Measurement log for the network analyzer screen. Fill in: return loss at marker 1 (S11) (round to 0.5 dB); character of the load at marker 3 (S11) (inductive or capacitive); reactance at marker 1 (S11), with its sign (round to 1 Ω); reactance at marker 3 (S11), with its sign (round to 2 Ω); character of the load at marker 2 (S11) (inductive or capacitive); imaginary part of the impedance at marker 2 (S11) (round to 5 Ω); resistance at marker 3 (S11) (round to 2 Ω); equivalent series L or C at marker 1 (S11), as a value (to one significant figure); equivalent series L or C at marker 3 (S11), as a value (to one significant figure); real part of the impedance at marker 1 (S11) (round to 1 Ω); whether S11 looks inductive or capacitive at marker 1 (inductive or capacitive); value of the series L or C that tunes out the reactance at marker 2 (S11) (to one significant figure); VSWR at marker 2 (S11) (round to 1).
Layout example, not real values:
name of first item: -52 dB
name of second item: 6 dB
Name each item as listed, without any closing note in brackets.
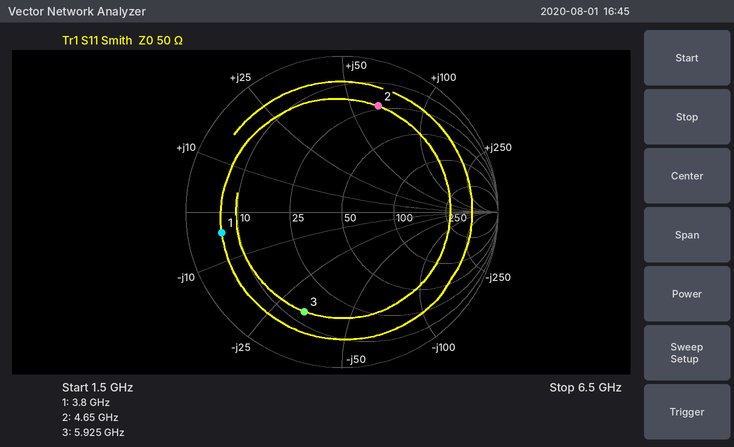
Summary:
return loss at marker 1 (S11): 2.0 dB
character of the load at marker 3 (S11): capacitive
reactance at marker 1 (S11), with its sign: -4 Ω
reactance at marker 3 (S11), with its sign: -32 Ω
character of the load at marker 2 (S11): inductive
imaginary part of the impedance at marker 2 (S11): +65 Ω
resistance at marker 3 (S11): 14 Ω
equivalent series L or C at marker 1 (S11), as a value: 10 pF
equivalent series L or C at marker 3 (S11), as a value: 800 fF
real part of the impedance at marker 1 (S11): 6 Ω
whether S11 looks inductive or capacitive at marker 1: capacitive
value of the series L or C that tunes out the reactance at marker 2 (S11): 500 fF
VSWR at marker 2 (S11): 6
